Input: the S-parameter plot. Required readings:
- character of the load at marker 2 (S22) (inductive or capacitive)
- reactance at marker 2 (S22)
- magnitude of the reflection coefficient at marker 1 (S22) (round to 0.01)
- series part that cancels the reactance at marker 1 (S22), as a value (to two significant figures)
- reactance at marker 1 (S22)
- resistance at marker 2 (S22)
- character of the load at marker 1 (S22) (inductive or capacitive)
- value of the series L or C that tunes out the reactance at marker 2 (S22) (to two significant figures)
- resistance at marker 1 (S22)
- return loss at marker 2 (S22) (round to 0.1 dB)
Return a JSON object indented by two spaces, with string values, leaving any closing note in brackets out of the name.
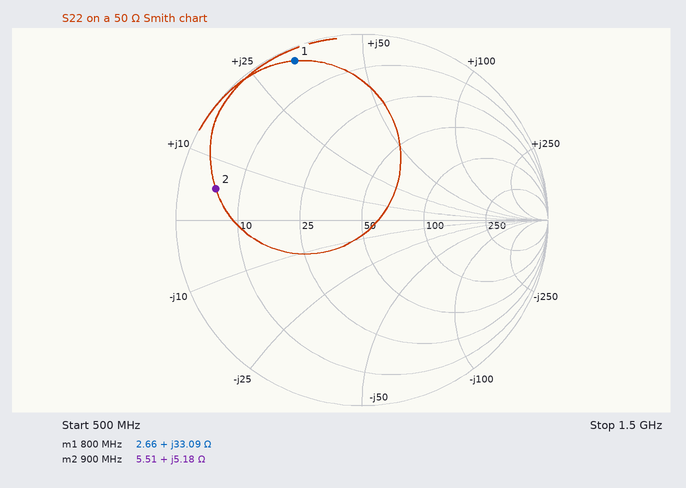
{
  "character of the load at marker 2 (S22)": "inductive",
  "reactance at marker 2": "+5.18 Ω",
  "magnitude of the reflection coefficient at marker 1 (S22)": "0.93",
  "series part that cancels the reactance at marker 1 (S22), as a value": "6.0 pF",
  "reactance at marker 1": "+33.09 Ω",
  "resistance at marker 2": "5.51 Ω",
  "character of the load at marker 1 (S22)": "inductive",
  "value of the series L or C that tunes out the reactance at marker 2 (S22)": "34 pF",
  "resistance at marker 1": "2.66 Ω",
  "return loss at marker 2 (S22)": "1.9 dB"
}
